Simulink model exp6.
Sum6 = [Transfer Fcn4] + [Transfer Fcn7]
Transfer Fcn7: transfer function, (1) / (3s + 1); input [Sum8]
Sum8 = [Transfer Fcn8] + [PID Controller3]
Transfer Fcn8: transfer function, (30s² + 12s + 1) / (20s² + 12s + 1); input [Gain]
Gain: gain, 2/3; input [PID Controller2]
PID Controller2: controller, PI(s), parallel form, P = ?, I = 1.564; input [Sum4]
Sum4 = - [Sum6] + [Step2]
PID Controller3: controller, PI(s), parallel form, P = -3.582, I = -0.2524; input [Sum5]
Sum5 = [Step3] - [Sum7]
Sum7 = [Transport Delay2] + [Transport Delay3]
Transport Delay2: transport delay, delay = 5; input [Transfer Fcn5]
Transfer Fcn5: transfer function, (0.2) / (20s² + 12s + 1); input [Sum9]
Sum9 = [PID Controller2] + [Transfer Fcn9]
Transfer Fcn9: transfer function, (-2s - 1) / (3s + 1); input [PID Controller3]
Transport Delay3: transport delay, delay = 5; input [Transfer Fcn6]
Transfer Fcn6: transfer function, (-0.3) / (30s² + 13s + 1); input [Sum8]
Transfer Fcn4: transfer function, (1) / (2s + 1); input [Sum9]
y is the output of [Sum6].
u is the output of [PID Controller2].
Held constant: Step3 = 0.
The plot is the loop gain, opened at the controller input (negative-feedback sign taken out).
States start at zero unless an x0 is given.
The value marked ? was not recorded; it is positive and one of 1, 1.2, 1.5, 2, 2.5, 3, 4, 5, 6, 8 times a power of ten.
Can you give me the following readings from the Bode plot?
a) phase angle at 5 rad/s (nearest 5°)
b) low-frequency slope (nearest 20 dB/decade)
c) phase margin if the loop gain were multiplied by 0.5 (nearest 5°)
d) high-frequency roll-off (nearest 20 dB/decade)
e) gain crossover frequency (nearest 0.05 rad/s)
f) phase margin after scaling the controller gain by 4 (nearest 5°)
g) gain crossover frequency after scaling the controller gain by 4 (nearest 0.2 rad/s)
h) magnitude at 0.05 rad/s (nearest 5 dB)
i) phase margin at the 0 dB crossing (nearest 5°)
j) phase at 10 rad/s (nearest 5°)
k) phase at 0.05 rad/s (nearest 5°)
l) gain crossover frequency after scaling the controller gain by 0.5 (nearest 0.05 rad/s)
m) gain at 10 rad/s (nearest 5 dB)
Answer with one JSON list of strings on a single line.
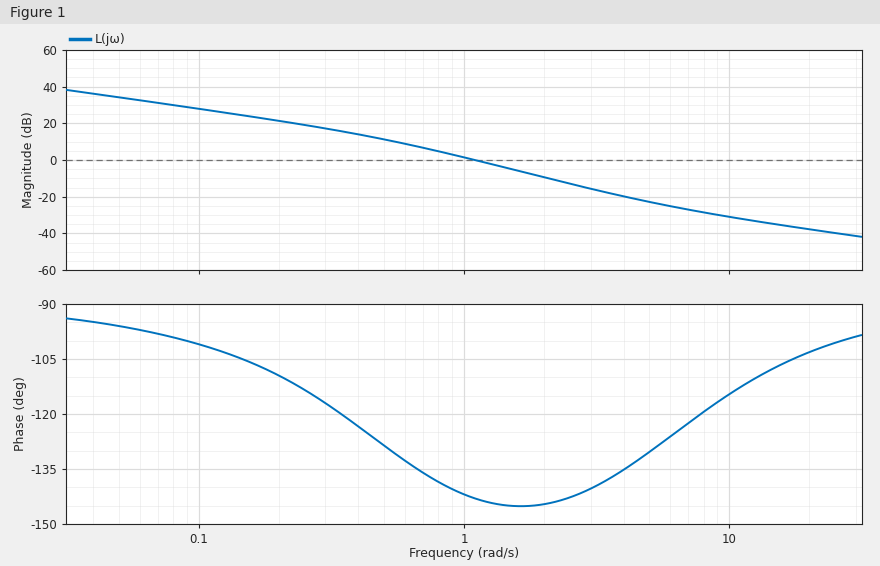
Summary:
["-130°", "-20 dB/decade", "45°", "-20 dB/decade", "1.10 rad/s", "35°", "2.4 rad/s", "35 dB", "35°", "-115°", "-95°", "0.75 rad/s", "-30 dB"]
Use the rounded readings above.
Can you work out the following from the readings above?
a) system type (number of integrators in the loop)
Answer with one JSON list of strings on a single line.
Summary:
["1"]
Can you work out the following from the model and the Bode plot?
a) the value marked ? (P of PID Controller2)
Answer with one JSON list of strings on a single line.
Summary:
["0.3"]
